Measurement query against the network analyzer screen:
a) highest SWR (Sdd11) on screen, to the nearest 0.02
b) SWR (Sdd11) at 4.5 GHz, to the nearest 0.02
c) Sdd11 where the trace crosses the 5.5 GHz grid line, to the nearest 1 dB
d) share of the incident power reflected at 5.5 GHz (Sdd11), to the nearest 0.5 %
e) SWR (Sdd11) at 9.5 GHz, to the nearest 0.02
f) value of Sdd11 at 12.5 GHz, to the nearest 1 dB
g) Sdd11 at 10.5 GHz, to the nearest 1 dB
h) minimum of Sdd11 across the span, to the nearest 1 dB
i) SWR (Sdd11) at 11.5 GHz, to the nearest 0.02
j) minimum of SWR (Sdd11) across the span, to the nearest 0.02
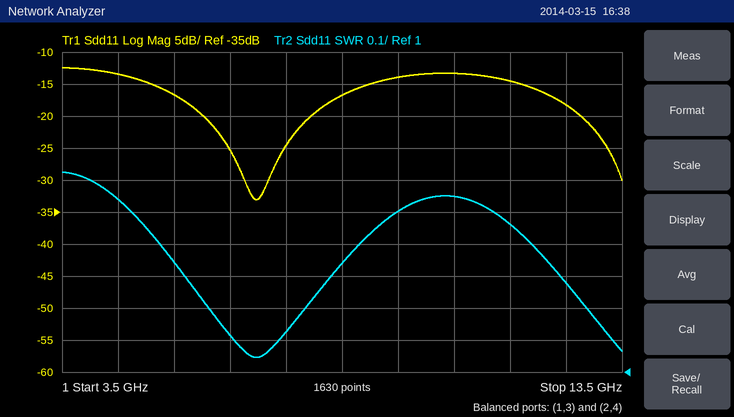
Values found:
1.62
1.54
-17 dB
2.0 %
1.50
-18 dB
-13 dB
-33 dB
1.46
1.04
